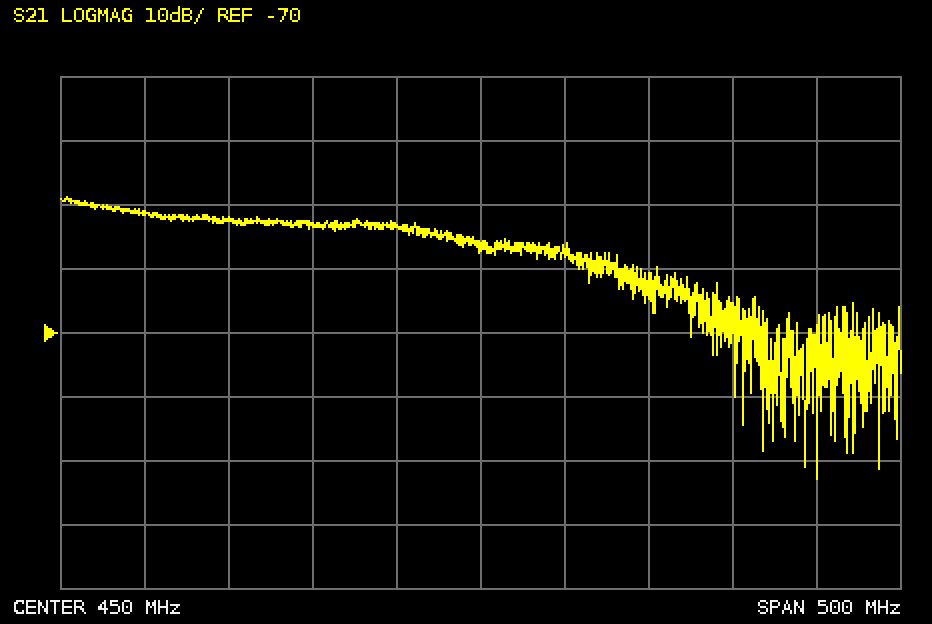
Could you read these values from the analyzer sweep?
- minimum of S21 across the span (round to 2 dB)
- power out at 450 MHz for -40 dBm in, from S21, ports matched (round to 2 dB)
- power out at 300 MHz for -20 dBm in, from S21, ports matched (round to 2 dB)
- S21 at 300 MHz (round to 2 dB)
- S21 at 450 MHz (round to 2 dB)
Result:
-92 dB
-96 dBm
-72 dBm
-52 dB
-56 dB
